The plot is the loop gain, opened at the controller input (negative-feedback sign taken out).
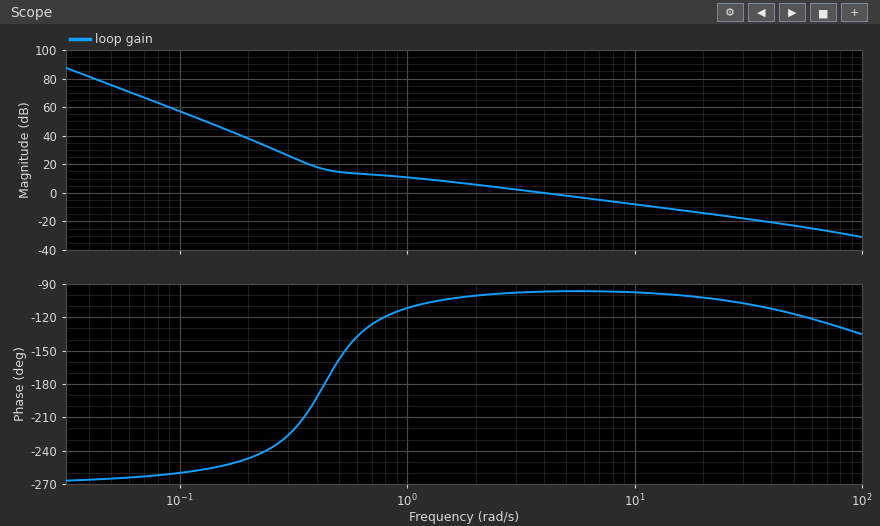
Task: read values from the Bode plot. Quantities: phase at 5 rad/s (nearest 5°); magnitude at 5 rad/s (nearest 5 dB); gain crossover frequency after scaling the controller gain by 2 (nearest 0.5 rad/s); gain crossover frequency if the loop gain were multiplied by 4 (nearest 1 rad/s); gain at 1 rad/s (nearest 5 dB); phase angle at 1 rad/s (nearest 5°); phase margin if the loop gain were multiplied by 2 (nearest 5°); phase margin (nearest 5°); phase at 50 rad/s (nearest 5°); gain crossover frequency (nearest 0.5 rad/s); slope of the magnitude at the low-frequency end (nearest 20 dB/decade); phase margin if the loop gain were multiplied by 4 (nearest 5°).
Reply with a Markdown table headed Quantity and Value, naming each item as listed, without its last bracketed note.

| Quantity | Value |
|---|---|
| phase at 5 rad/s | -95° |
| magnitude at 5 rad/s | 0 dB |
| gain crossover frequency after scaling the controller gain by 2 | 8.0 rad/s |
| gain crossover frequency if the loop gain were multiplied by 4 | 16 rad/s |
| gain at 1 rad/s | 10 dB |
| phase angle at 1 rad/s | -110° |
| phase margin if the loop gain were multiplied by 2 | 85° |
| phase margin | 85° |
| phase at 50 rad/s | -115° |
| gain crossover frequency | 4.0 rad/s |
| slope of the magnitude at the low-frequency end | -60 dB/decade |
| phase margin if the loop gain were multiplied by 4 | 80° |
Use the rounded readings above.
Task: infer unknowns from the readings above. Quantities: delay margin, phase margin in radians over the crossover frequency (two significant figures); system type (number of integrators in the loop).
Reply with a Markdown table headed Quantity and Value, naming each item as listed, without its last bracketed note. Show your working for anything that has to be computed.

| Quantity | Value |
|---|---|
| delay margin, phase margin in radians over the crossover frequency | 85 × π / 180 / 4 = 0.37 s |
| system type | 3 |
